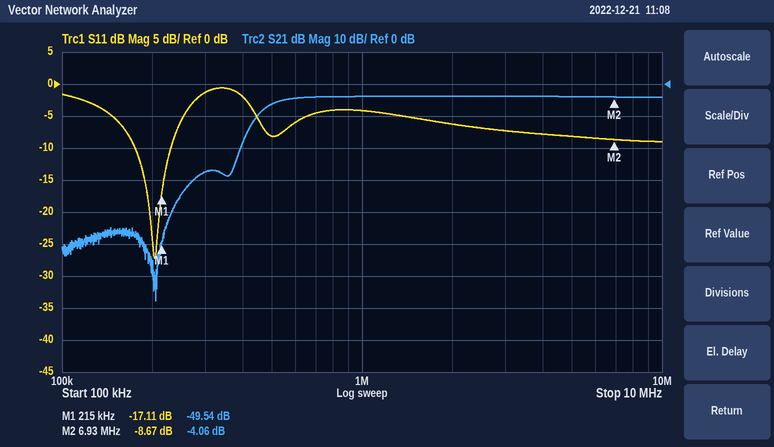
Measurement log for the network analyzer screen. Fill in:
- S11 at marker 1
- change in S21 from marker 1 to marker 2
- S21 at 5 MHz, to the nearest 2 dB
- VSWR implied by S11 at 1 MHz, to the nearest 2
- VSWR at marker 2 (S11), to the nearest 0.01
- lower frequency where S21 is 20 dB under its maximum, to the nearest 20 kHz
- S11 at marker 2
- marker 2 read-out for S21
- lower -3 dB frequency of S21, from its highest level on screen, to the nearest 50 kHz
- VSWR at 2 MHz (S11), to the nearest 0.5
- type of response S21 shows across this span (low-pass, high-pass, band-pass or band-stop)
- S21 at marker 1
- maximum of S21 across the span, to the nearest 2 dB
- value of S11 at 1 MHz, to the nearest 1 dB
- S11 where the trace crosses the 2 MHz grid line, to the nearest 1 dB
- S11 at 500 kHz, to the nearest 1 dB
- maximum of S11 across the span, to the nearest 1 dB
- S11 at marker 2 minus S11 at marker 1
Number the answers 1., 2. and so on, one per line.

1. -17.11 dB
2. 45.48 dB
3. -4 dB
4. 4
5. 2.17
6. 380 kHz
7. -8.67 dB
8. -4.06 dB
9. 500 kHz
10. 3.0
11. high-pass
12. -49.54 dB
13. -4 dB
14. -4 dB
15. -6 dB
16. -8 dB
17. -1 dB
18. 8.44 dB
